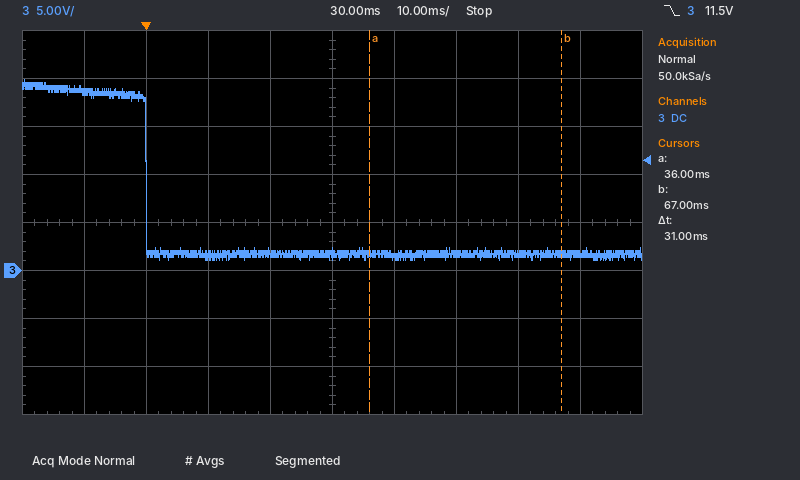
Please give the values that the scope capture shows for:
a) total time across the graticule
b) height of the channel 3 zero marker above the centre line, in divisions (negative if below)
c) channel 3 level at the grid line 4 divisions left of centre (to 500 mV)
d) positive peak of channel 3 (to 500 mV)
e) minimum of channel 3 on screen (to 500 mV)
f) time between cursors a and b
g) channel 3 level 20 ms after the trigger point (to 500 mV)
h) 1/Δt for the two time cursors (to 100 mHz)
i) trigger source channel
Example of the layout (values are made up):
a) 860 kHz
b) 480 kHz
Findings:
a) 100 ms
b) -1.0 div
c) 18.5 V
d) 20.0 V
e) 1.0 V
f) 31 ms
g) 2.0 V
h) 32.3 Hz
i) channel 3
